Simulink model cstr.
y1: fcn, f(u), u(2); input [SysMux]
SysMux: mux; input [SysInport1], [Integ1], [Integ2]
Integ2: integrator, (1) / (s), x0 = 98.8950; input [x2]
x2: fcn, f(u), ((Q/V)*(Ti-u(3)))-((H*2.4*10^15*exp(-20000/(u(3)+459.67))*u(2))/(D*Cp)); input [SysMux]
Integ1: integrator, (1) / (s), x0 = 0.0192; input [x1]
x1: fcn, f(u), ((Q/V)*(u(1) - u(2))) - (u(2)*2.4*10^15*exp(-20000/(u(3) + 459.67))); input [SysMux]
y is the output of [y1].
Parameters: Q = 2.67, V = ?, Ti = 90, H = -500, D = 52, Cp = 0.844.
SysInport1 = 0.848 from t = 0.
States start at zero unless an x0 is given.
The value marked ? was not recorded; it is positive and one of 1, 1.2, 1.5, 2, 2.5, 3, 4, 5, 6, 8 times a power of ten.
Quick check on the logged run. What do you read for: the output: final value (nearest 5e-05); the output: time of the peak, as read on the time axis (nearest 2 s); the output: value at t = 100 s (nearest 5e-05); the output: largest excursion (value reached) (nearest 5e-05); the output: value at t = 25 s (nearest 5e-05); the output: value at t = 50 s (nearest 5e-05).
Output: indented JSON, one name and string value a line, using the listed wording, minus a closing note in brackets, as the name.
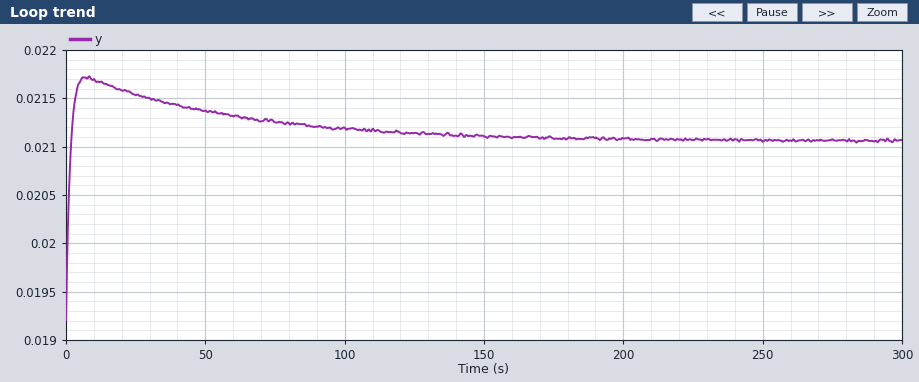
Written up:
{
  "the output: final value": "0.02105",
  "the output: time of the peak, as read on the time axis": "8 s",
  "the output: value at t = 100 s": "0.02120",
  "the output: largest excursion (value reached)": "0.02170",
  "the output: value at t = 25 s": "0.02155",
  "the output: value at t = 50 s": "0.02135"
}
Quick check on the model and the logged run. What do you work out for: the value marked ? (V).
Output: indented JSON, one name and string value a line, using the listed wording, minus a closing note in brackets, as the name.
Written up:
{
  "the value marked ?": "150"
}
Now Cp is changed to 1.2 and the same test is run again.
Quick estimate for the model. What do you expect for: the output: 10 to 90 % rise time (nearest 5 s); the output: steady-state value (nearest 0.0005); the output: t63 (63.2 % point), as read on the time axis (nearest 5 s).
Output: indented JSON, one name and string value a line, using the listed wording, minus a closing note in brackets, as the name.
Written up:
{
  "the output: 10 to 90 % rise time": "100 s",
  "the output: steady-state value": "0.0250",
  "the output: t63 (63.2 % point), as read on the time axis": "25 s"
}
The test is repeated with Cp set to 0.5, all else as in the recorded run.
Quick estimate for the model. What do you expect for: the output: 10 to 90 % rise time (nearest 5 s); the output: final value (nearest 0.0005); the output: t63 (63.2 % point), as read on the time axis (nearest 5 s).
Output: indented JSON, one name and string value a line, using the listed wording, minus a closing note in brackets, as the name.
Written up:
{
  "the output: 10 to 90 % rise time": "115 s",
  "the output: final value": "0.0140",
  "the output: t63 (63.2 % point), as read on the time axis": "70 s"
}
